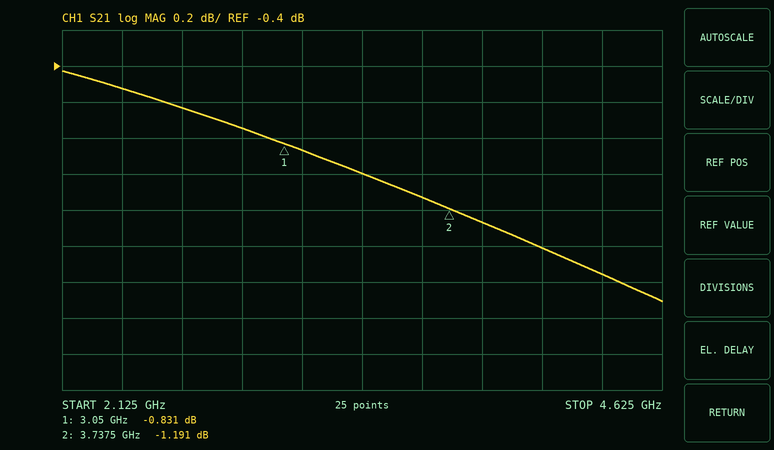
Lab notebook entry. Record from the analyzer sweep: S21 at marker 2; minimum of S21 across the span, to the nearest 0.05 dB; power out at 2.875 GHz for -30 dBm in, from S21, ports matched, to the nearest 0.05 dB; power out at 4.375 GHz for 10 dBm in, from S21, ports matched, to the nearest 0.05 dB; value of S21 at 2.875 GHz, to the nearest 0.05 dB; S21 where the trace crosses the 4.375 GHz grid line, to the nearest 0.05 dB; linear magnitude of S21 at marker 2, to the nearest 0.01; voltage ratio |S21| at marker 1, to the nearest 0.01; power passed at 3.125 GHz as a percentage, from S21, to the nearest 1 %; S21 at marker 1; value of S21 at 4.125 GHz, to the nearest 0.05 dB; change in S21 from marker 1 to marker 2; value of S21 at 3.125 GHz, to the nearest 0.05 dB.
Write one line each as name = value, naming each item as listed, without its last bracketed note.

S21 at marker 2 = -1.191 dB
minimum of S21 across the span, to the nearest 0.05 dB = -1.70 dB
power out at 2.875 GHz for -30 dBm in, from S21, ports matched, to the nearest 0.05 dB = -30.75 dBm
power out at 4.375 GHz for 10 dBm in, from S21, ports matched, to the nearest 0.05 dB = 8.45 dBm
value of S21 at 2.875 GHz, to the nearest 0.05 dB = -0.75 dB
S21 where the trace crosses the 4.375 GHz grid line, to the nearest 0.05 dB = -1.55 dB
linear magnitude of S21 at marker 2, to the nearest 0.01 = 0.87
voltage ratio |S21| at marker 1, to the nearest 0.01 = 0.91
power passed at 3.125 GHz as a percentage, from S21, to the nearest 1 % = 82 %
S21 at marker 1 = -0.831 dB
value of S21 at 4.125 GHz, to the nearest 0.05 dB = -1.40 dB
change in S21 from marker 1 to marker 2 = -0.360 dB
value of S21 at 3.125 GHz, to the nearest 0.05 dB = -0.85 dB
